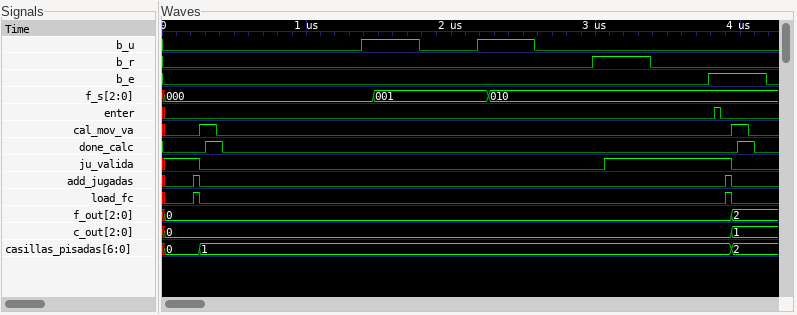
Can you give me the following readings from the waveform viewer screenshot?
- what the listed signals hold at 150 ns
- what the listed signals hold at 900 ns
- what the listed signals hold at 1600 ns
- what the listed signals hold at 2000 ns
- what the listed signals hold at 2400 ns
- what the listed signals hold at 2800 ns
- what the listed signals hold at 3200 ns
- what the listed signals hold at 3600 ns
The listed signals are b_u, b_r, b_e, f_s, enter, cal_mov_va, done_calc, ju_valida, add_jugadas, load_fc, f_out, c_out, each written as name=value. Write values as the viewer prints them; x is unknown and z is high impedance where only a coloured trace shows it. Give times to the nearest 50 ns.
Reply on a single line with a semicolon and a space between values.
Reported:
b_u=0, b_r=0, b_e=0, f_s=000, enter=0, cal_mov_va=0, done_calc=0, ju_valida=1, add_jugadas=0, load_fc=0, f_out=0, c_out=0; b_u=0, b_r=0, b_e=0, f_s=000, enter=0, cal_mov_va=0, done_calc=0, ju_valida=0, add_jugadas=0, load_fc=0, f_out=0, c_out=0; b_u=1, b_r=0, b_e=0, f_s=001, enter=0, cal_mov_va=0, done_calc=0, ju_valida=0, add_jugadas=0, load_fc=0, f_out=0, c_out=0; b_u=0, b_r=0, b_e=0, f_s=001, enter=0, cal_mov_va=0, done_calc=0, ju_valida=0, add_jugadas=0, load_fc=0, f_out=0, c_out=0; b_u=1, b_r=0, b_e=0, f_s=010, enter=0, cal_mov_va=0, done_calc=0, ju_valida=0, add_jugadas=0, load_fc=0, f_out=0, c_out=0; b_u=0, b_r=0, b_e=0, f_s=010, enter=0, cal_mov_va=0, done_calc=0, ju_valida=0, add_jugadas=0, load_fc=0, f_out=0, c_out=0; b_u=0, b_r=1, b_e=0, f_s=010, enter=0, cal_mov_va=0, done_calc=0, ju_valida=1, add_jugadas=0, load_fc=0, f_out=0, c_out=0; b_u=0, b_r=0, b_e=0, f_s=010, enter=0, cal_mov_va=0, done_calc=0, ju_valida=1, add_jugadas=0, load_fc=0, f_out=0, c_out=0
